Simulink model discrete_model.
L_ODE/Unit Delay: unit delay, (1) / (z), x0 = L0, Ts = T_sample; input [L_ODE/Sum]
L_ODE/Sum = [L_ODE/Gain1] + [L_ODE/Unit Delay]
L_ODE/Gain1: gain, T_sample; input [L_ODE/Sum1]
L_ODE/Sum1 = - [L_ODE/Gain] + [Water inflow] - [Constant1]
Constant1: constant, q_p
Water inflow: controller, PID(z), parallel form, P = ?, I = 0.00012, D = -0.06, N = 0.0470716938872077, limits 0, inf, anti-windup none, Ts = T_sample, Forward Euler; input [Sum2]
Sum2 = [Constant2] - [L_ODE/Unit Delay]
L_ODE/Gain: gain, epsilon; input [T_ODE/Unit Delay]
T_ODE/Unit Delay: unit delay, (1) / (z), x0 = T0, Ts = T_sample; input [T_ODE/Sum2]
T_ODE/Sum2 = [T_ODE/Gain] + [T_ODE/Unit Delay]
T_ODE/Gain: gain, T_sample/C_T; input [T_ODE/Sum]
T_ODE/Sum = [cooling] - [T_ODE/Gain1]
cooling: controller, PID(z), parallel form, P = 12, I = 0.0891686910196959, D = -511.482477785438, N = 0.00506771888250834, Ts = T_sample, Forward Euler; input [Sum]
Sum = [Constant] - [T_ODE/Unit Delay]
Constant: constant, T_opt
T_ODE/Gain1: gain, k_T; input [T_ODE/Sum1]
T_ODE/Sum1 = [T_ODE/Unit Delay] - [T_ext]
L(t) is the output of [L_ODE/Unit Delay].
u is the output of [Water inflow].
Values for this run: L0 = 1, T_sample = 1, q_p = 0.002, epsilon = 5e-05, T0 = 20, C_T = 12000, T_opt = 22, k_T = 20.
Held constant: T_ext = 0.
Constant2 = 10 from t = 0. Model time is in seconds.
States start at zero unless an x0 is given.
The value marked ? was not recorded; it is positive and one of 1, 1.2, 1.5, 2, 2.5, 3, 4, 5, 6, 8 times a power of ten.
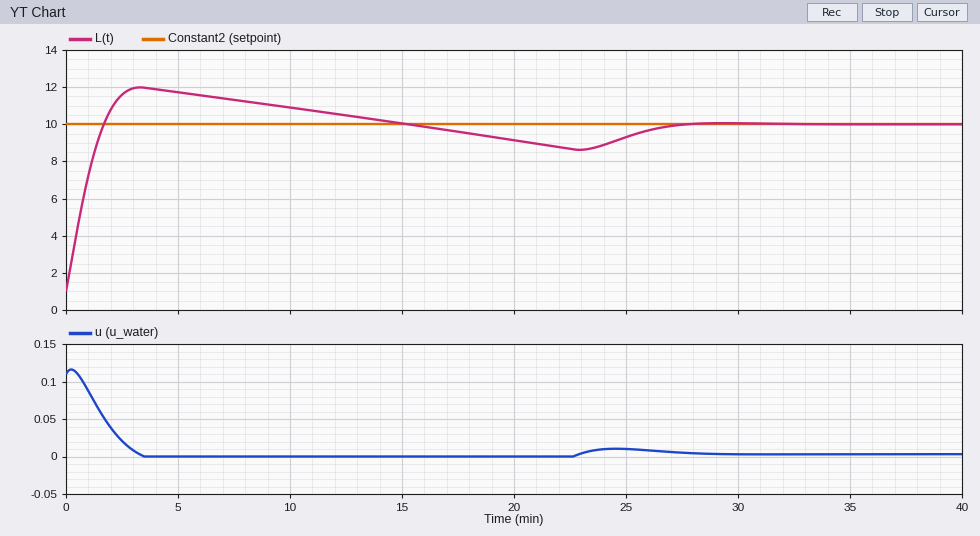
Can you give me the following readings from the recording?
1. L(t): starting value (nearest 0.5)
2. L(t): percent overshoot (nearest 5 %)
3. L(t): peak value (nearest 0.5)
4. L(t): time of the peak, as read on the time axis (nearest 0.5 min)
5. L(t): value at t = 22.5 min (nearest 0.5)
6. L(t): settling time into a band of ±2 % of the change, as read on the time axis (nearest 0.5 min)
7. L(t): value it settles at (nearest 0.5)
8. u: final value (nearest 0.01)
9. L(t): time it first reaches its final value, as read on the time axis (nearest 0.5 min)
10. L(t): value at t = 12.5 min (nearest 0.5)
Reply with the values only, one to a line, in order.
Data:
1.0
20 %
12.0
3.5 min
8.5
26.5 min
10.0
0.00
1.5 min
10.5
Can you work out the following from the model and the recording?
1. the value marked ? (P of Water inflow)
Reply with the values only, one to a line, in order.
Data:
0.015
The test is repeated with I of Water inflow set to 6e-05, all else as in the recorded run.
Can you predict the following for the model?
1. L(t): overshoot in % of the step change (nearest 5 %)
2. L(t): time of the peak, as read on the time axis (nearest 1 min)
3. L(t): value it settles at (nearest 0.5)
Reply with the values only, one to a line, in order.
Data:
15 %
4 min
10.0
